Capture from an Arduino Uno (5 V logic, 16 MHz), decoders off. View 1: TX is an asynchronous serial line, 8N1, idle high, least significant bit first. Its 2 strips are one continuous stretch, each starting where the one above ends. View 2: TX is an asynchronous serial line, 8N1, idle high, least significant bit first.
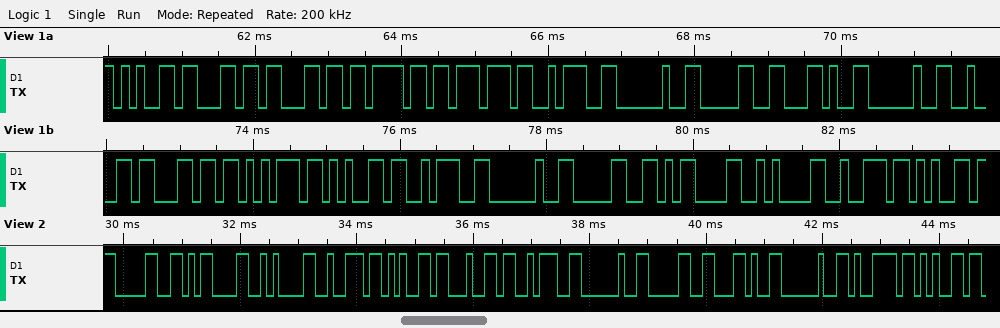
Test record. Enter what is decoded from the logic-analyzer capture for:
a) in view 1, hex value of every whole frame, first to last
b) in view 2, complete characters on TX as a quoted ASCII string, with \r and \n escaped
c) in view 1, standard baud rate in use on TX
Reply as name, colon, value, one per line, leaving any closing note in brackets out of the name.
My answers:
in view 1, hex value of every whole frame, first to last: 65 6C 6C 6F 77 3A 20 30 2C 20 62 6C 75 65 3A 20 30 0D 0A 72 65
in view 2, complete characters on TX as a quoted ASCII string, with \r and \n escaped: "0\r\nred: 0, ye"
in view 1, standard baud rate in use on TX: 9600 baud
